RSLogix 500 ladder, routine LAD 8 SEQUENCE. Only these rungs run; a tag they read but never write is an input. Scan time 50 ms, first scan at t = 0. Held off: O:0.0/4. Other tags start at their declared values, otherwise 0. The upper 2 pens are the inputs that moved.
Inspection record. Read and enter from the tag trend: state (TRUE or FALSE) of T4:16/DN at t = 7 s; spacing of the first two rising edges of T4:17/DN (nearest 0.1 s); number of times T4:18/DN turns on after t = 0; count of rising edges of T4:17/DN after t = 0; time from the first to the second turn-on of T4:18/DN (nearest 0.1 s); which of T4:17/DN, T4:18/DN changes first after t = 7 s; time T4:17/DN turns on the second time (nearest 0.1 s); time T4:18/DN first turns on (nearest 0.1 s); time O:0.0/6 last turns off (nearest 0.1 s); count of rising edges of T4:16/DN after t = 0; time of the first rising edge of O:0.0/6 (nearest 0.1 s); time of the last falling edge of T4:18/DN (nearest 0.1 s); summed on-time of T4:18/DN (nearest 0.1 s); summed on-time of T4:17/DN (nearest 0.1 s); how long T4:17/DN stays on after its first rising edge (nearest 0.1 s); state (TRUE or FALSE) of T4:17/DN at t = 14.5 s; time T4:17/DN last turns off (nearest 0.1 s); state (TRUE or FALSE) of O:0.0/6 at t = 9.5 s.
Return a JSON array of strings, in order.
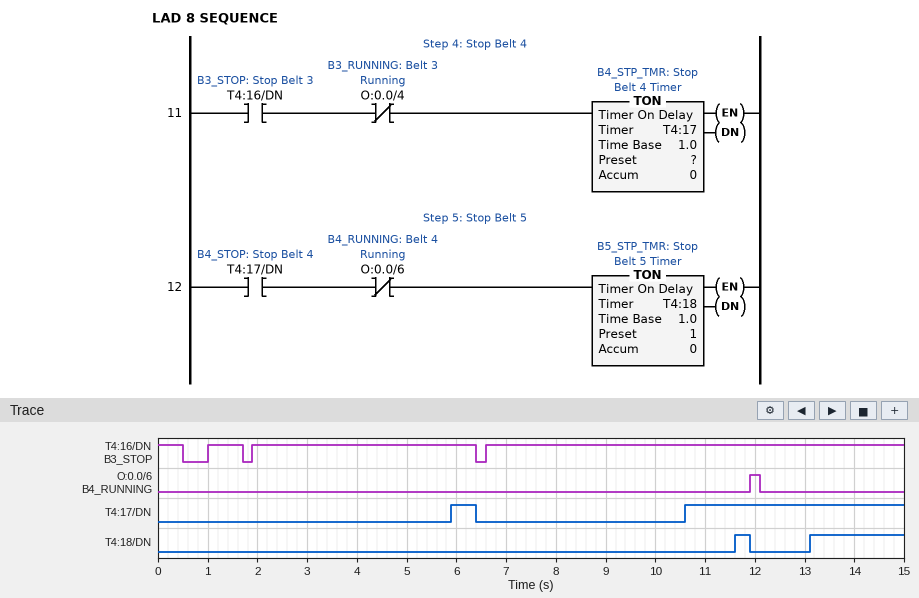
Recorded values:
["TRUE", "4.7 s", "2", "2", "1.5 s", "T4:17/DN", "10.6 s", "11.6 s", "12.1 s", "3", "11.9 s", "11.9 s", "2.2 s", "4.9 s", "0.5 s", "TRUE", "6.4 s", "FALSE"]
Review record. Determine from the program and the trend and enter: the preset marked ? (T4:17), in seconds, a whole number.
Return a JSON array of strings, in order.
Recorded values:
["4 s"]
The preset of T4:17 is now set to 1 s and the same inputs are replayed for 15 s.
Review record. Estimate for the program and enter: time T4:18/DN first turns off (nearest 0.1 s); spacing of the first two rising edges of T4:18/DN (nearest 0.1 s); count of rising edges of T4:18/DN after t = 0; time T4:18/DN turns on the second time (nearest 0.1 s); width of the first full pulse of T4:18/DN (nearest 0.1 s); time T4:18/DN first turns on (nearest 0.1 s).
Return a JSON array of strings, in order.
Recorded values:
["6.4 s", "4.7 s", "3", "8.6 s", "2.5 s", "3.9 s"]
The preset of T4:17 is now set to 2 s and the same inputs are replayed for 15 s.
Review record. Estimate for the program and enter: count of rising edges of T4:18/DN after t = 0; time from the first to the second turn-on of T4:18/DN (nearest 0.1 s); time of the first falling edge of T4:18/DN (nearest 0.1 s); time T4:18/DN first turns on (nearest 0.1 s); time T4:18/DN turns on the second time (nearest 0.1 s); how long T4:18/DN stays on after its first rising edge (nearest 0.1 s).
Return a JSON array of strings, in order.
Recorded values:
["3", "4.7 s", "6.4 s", "4.9 s", "9.6 s", "1.5 s"]
